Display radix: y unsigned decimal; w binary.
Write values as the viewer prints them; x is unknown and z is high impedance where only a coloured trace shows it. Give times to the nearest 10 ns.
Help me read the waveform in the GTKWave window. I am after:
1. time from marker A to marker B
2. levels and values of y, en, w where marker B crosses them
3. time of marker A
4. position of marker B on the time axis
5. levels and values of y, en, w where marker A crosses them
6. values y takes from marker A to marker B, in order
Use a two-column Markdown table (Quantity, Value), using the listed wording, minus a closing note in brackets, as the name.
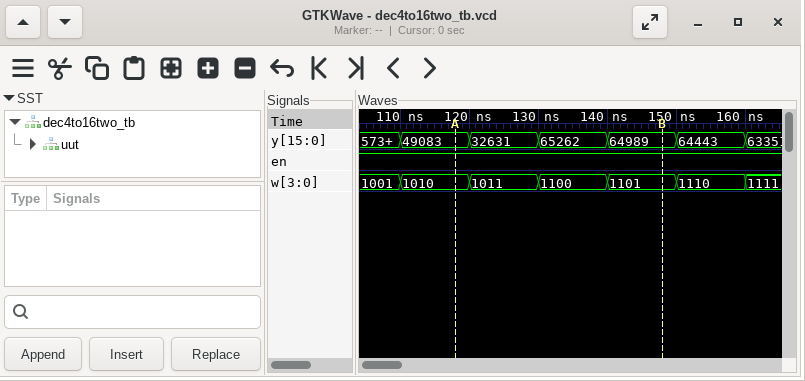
| Quantity | Value |
|---|---|
| time from marker A to marker B | 30 ns |
| levels and values of y, en, w where marker B crosses them | y=64989, en=1, w=1101 |
| time of marker A | 120 ns |
| position of marker B on the time axis | 150 ns |
| levels and values of y, en, w where marker A crosses them | y=49083, en=1, w=1010 |
| values y takes from marker A to marker B, in order | 49083, 32631, 65262, 64989 |
